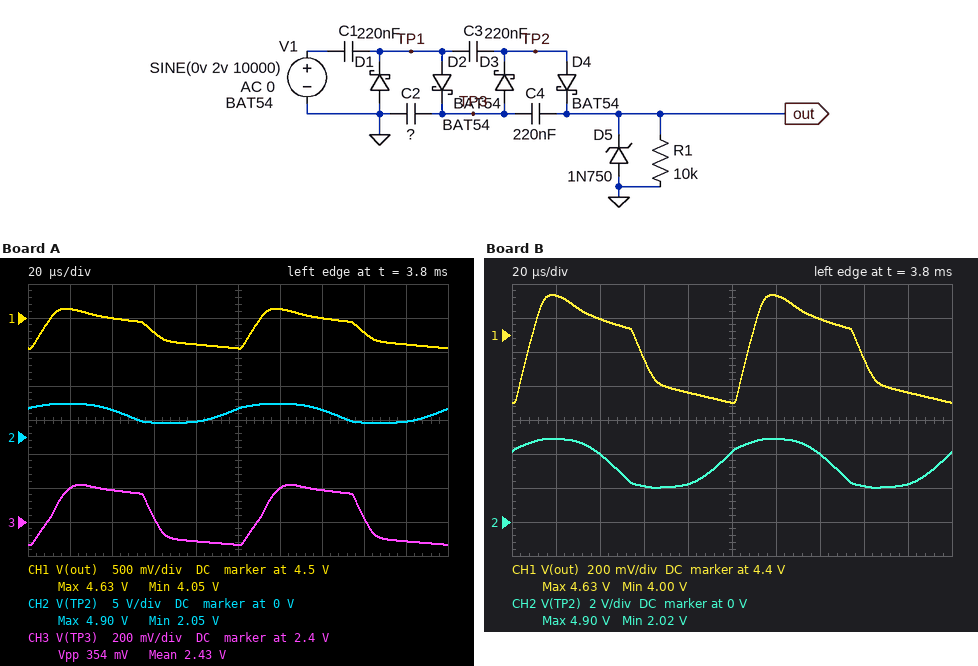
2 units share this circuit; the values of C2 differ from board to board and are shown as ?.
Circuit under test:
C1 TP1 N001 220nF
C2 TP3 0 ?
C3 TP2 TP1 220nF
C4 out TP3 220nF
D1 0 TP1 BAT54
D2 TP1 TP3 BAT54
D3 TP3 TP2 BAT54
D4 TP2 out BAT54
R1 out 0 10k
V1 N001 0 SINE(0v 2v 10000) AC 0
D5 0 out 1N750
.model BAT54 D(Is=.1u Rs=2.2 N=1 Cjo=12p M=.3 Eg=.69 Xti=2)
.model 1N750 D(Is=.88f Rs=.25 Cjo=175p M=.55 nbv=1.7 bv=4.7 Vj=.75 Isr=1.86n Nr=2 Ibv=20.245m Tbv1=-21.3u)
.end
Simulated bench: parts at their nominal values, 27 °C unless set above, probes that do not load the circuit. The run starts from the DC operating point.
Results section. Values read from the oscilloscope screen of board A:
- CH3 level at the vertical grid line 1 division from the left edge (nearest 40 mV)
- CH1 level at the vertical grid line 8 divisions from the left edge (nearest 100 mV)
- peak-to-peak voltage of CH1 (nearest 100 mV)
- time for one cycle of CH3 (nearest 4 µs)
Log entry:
2.60 V
4.3 V
600 mV
100 µs
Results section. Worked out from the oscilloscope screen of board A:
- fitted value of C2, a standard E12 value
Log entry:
390 nF
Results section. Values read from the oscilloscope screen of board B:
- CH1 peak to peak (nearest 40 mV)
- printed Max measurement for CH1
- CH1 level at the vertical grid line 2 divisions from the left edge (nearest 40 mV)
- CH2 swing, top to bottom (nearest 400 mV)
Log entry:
640 mV
4.63 V
4.48 V
2.8 V
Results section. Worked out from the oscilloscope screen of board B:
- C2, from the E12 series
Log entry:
330 nF
